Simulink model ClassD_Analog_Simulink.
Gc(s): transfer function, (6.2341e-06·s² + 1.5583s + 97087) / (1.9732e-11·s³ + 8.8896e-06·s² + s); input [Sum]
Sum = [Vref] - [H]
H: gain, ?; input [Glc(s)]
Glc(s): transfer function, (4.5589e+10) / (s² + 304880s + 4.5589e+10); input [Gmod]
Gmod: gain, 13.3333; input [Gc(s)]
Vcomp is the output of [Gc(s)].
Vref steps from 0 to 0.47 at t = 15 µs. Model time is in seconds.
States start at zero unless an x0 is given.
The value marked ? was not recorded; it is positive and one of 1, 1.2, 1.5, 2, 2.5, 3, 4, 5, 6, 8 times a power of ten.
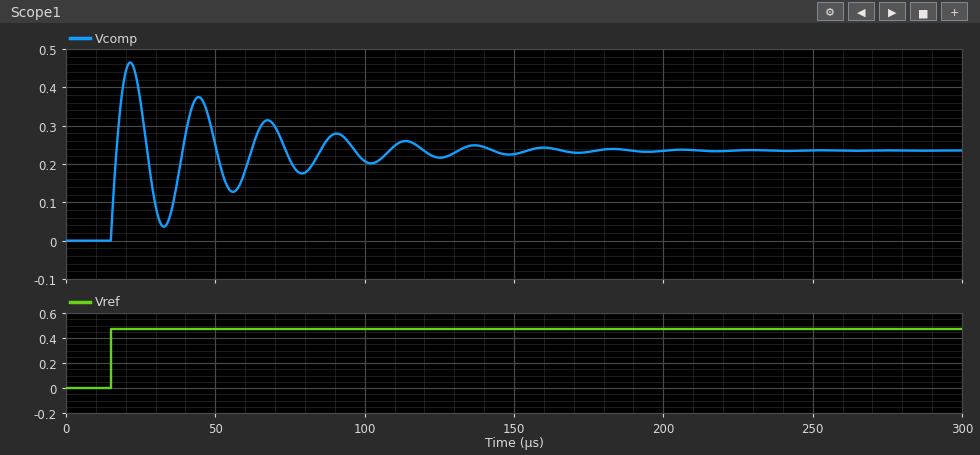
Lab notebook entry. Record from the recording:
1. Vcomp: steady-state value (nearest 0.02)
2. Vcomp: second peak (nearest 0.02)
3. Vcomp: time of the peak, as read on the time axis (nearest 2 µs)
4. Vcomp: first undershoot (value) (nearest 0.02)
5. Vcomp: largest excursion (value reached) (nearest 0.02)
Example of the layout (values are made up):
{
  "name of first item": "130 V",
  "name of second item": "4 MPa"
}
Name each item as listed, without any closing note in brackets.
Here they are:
{
  "Vcomp: steady-state value": "0.24",
  "Vcomp: second peak": "0.38",
  "Vcomp: time of the peak, as read on the time axis": "22 µs",
  "Vcomp: first undershoot (value)": "0.04",
  "Vcomp: largest excursion (value reached)": "0.46"
}
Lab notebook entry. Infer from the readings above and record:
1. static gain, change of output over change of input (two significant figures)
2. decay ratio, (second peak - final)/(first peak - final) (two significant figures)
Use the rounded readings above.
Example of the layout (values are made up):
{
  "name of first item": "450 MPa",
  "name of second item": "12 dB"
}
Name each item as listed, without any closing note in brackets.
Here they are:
{
  "static gain, change of output over change of input": "0.51",
  "decay ratio, (second peak - final)/(first peak - final)": "0.64"
}
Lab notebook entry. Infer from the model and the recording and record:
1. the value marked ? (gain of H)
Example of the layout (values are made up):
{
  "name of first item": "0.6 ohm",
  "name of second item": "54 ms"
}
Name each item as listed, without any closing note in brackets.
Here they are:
{
  "the value marked ?": "0.15"
}
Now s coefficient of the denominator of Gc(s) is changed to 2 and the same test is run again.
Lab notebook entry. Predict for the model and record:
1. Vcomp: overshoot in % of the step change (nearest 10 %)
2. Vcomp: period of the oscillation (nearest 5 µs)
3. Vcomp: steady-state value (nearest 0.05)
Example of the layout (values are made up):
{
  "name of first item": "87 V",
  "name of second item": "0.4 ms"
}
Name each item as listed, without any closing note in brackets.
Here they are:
{
  "Vcomp: overshoot in % of the step change": "60 %",
  "Vcomp: period of the oscillation": "20 µs",
  "Vcomp: steady-state value": "0.25"
}
